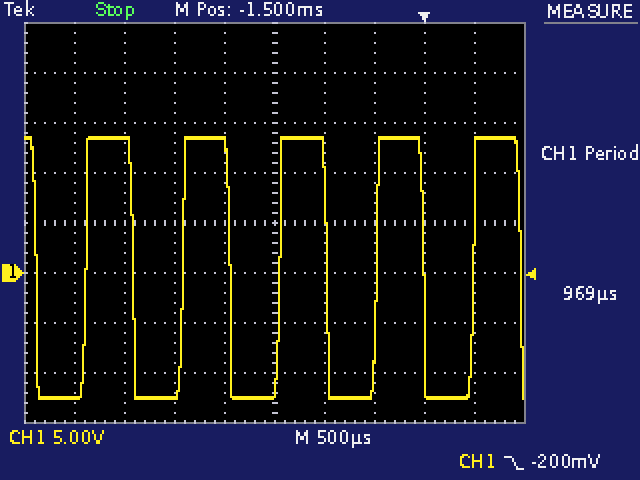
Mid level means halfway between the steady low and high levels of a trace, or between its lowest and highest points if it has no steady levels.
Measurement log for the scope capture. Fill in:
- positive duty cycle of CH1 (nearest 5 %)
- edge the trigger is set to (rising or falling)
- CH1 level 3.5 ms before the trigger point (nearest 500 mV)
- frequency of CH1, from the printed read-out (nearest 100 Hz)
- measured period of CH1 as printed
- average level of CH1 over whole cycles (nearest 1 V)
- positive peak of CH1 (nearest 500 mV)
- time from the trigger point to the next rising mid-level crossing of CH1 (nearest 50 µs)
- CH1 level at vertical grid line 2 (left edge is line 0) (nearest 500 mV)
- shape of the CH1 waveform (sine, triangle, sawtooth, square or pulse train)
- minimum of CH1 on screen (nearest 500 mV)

50 %
falling
-12.5 V
1.0 kHz
969 µs
0 V
13.5 V
500 µs
13.5 V
square
-12.5 V
